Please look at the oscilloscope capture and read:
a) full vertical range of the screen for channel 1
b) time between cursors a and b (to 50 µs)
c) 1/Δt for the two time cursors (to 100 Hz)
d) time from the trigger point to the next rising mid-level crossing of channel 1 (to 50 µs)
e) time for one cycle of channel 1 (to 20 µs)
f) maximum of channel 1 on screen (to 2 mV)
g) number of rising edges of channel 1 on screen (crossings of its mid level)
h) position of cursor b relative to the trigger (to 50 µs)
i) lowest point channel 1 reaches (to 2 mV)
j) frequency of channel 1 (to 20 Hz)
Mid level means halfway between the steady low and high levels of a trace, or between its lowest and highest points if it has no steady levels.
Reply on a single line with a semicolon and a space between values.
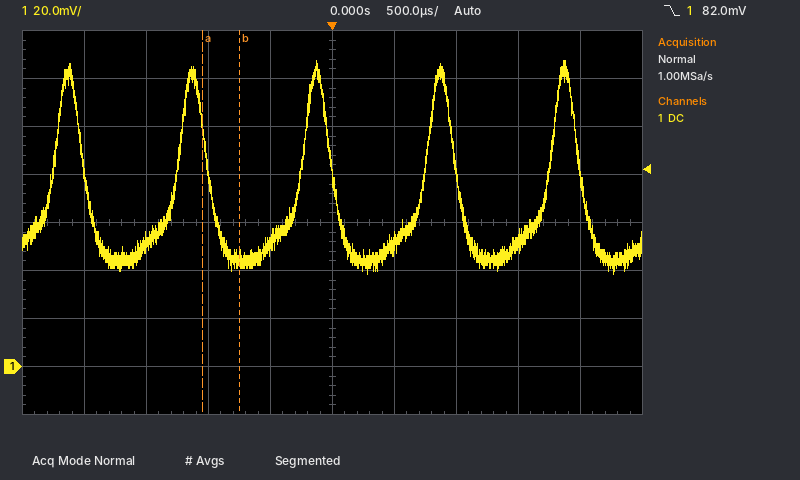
160 mV; 300 µs; 3.3 kHz; 750 µs; 1.00 ms; 128 mV; 5; -750 µs; 38 mV; 1.00 kHz
